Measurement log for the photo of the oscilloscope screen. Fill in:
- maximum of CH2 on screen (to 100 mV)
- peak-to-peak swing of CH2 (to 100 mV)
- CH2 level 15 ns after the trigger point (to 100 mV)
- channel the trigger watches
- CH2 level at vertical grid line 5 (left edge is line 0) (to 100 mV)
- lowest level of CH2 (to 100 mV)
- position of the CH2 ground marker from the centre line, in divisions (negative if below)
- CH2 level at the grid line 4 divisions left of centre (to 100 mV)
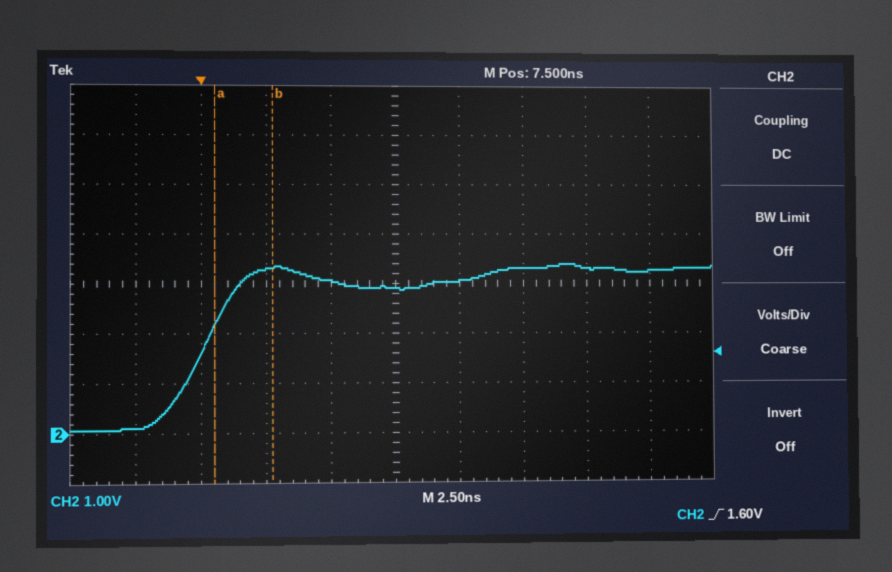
3.4 V
3.3 V
3.3 V
CH2
2.9 V
100 mV
-3.0 div
100 mV
